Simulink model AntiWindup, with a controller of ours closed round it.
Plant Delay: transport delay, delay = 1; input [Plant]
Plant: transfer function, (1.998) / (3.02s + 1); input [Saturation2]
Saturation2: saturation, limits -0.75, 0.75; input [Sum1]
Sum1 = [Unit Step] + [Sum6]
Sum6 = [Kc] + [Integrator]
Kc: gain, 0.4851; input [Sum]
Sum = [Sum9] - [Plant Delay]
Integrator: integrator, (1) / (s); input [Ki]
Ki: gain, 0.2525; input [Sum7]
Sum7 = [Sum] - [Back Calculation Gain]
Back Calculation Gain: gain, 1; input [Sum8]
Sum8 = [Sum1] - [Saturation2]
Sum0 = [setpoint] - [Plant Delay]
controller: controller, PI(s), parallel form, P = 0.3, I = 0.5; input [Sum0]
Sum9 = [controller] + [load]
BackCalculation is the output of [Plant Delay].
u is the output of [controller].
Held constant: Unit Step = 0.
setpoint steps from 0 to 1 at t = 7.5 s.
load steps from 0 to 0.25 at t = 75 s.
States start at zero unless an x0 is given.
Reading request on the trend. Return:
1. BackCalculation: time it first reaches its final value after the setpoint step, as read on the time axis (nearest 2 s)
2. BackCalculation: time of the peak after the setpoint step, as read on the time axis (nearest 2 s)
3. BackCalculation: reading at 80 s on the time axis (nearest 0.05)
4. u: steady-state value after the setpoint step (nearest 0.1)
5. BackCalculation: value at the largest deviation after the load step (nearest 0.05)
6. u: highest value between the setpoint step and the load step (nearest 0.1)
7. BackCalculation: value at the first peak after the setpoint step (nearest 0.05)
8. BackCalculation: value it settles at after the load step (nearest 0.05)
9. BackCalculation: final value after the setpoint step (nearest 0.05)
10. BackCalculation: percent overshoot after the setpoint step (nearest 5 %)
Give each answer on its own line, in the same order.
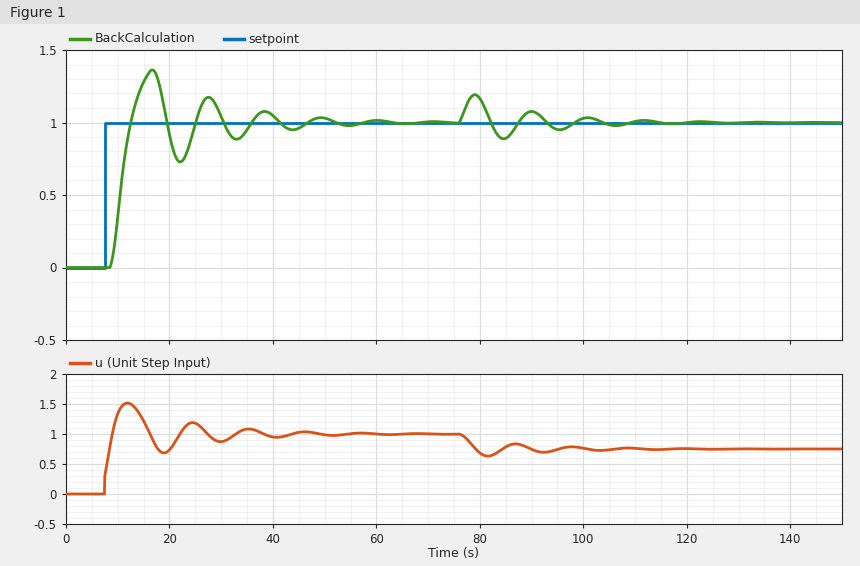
12 s
16 s
1.15
1.0
1.20
1.5
1.35
1.00
1.00
35 %
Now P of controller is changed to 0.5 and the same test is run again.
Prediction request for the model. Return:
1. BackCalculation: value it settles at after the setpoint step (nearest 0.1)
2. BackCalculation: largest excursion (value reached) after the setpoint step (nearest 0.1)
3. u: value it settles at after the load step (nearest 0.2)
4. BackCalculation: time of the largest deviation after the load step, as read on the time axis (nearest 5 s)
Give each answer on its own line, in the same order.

1.0
1.3
0.8
80 s
